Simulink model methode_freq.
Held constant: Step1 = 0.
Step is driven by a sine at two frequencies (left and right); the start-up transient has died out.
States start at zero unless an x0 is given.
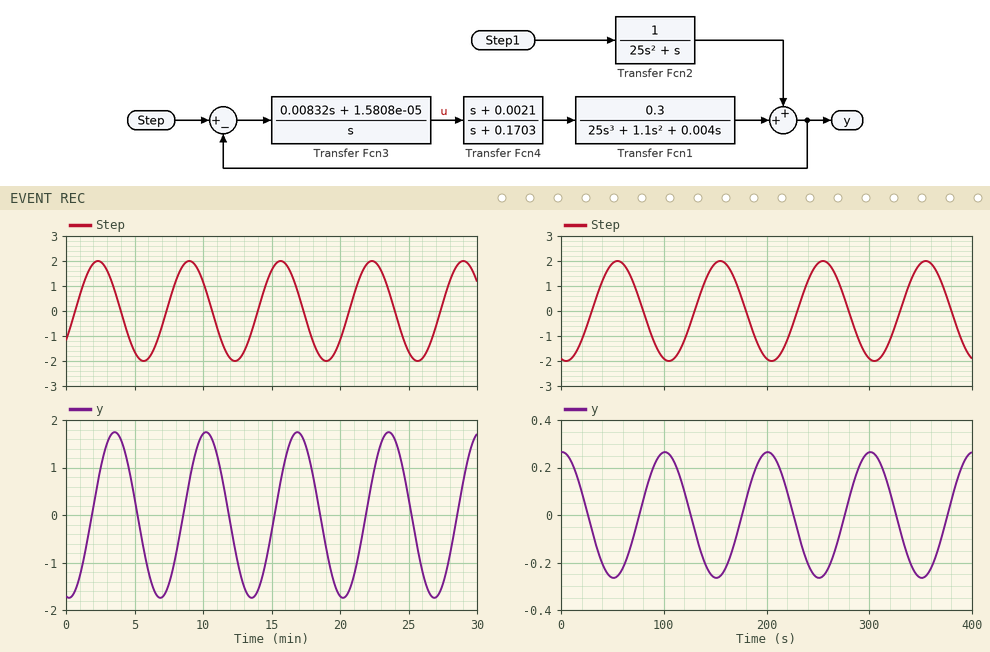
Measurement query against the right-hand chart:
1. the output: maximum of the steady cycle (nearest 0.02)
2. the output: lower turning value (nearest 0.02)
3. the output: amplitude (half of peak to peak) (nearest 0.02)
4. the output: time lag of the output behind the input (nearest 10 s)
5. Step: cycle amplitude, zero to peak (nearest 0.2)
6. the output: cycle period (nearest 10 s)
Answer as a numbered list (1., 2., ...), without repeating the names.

1. 0.26
2. -0.26
3. 0.26
4. 50 s
5. 2.0
6. 100 s
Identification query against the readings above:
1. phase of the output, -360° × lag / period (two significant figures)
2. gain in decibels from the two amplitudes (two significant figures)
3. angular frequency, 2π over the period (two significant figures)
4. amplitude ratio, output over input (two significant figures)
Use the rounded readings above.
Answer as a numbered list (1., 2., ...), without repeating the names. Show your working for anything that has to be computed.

1. -360 × 50 / 100 = -180°
2. 20 log10(0.26 / 2) = -18 dB
3. 2π / 100 = 0.063 rad/s
4. 0.26 / 2 = 0.13
